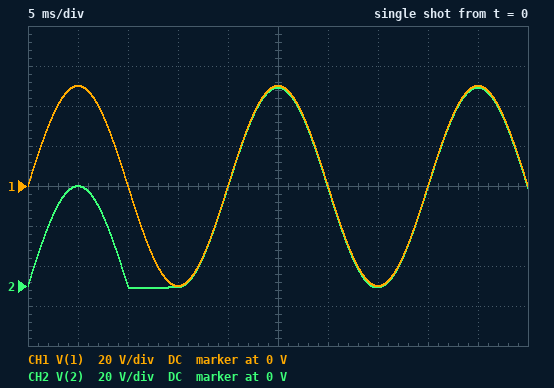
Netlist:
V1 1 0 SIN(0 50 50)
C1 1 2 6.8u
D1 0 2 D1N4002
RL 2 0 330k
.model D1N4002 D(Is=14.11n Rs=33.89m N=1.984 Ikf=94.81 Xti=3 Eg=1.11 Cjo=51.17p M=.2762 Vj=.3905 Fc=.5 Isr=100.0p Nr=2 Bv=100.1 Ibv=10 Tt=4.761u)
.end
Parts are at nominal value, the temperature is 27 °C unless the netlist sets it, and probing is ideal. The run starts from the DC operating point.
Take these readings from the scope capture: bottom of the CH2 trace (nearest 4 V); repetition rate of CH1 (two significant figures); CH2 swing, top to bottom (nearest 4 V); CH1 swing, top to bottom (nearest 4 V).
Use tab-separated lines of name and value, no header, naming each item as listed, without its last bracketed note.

bottom of the CH2 trace	0 V
repetition rate of CH1	50 Hz
CH2 swing, top to bottom	100 V
CH1 swing, top to bottom	100 V
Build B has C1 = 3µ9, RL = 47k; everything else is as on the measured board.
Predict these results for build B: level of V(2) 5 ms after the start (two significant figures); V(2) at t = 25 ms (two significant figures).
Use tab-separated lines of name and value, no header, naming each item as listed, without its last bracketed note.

level of V(2) 5 ms after the start	49 V
V(2) at t = 25 ms	97 V
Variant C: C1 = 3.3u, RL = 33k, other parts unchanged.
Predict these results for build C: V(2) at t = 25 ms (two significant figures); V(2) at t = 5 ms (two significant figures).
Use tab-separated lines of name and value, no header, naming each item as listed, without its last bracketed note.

V(2) at t = 25 ms	95 V
V(2) at t = 5 ms	49 V
